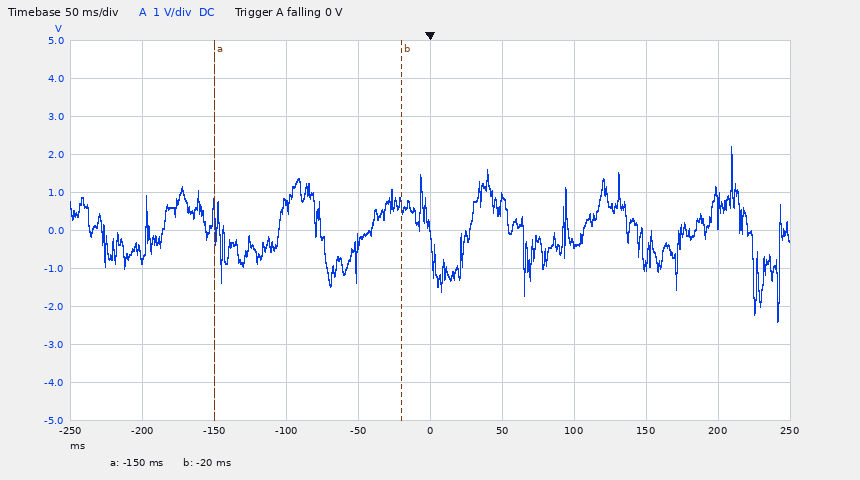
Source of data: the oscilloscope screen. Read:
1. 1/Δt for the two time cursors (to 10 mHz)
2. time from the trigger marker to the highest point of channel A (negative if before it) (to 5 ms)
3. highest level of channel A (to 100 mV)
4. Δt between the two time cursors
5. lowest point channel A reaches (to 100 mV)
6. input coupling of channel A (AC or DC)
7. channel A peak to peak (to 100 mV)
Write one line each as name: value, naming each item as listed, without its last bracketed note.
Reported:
1/Δt for the two time cursors: 7.69 Hz
time from the trigger marker to the highest point of channel A (negative if before it): +210 ms
highest level of channel A: 2.2 V
Δt between the two time cursors: 130 ms
lowest point channel A reaches: -2.4 V
input coupling of channel A: DC
channel A peak to peak: 4.6 V
